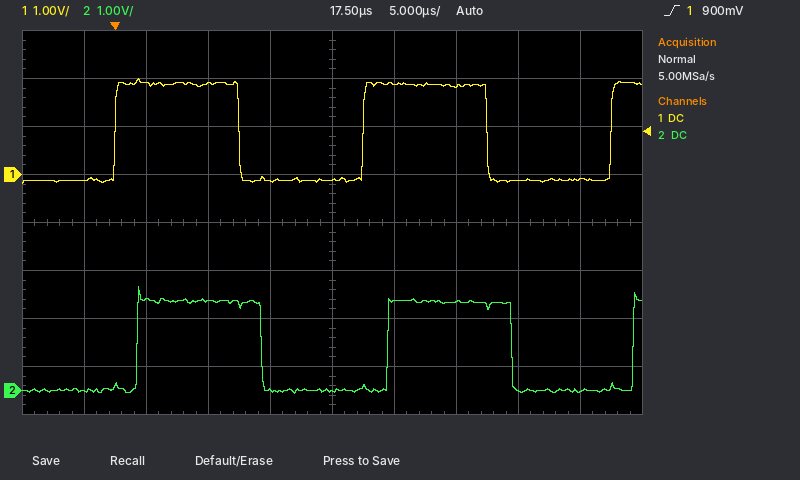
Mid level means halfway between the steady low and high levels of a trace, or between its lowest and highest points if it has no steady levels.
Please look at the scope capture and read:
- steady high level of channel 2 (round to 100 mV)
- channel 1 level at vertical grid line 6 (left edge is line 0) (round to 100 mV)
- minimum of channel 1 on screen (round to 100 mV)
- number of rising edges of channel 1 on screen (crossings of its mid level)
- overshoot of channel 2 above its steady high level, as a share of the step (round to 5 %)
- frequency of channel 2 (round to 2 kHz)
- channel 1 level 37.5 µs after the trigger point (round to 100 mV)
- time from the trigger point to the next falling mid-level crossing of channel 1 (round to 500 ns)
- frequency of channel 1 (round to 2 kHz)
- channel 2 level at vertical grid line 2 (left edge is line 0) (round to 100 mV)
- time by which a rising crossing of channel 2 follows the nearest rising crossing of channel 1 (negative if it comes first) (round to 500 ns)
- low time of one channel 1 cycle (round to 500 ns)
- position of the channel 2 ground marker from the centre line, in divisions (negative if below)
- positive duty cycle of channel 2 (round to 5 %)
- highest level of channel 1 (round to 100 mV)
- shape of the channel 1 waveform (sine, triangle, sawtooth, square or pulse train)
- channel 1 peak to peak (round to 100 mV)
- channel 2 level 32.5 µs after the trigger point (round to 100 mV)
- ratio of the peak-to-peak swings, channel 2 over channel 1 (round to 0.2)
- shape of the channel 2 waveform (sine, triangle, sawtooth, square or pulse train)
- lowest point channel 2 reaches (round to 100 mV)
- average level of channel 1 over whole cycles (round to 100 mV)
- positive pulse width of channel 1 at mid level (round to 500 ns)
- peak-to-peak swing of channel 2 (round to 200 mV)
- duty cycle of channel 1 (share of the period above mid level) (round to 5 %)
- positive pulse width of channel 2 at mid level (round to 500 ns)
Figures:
1.9 V
1.9 V
-200 mV
3
15 %
50 kHz
-100 mV
10.0 µs
50 kHz
1.9 V
+2.0 µs
10.0 µs
-3.5 div
50 %
2.0 V
square
2.2 V
0.0 V
1.0
square
-100 mV
900 mV
10.0 µs
2.2 V
50 %
10.0 µs
